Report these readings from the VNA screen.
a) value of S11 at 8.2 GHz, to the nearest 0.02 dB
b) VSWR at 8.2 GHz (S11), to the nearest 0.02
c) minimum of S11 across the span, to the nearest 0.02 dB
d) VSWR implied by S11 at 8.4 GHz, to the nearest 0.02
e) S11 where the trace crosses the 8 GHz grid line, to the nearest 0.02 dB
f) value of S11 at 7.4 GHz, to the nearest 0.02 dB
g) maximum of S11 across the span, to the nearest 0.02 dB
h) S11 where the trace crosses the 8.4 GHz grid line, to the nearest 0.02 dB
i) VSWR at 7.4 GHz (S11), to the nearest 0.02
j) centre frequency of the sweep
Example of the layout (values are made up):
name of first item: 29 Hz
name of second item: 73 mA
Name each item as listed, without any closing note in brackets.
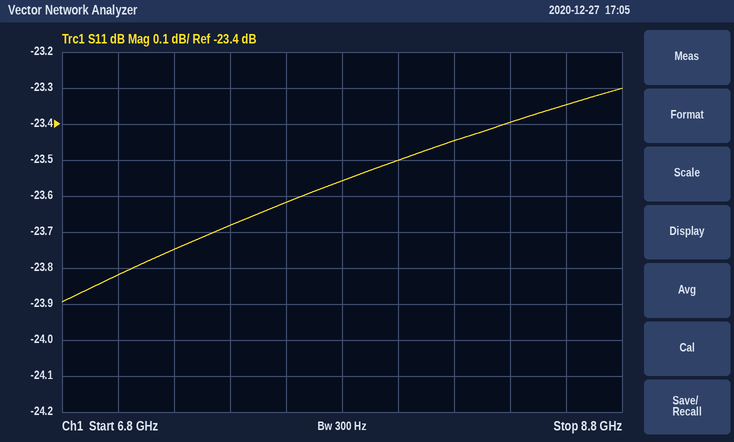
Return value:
value of S11 at 8.2 GHz, to the nearest 0.02 dB: -23.44 dB
VSWR at 8.2 GHz (S11), to the nearest 0.02: 1.14
minimum of S11 across the span, to the nearest 0.02 dB: -23.90 dB
VSWR implied by S11 at 8.4 GHz, to the nearest 0.02: 1.14
S11 where the trace crosses the 8 GHz grid line, to the nearest 0.02 dB: -23.50 dB
value of S11 at 7.4 GHz, to the nearest 0.02 dB: -23.68 dB
maximum of S11 across the span, to the nearest 0.02 dB: -23.30 dB
S11 where the trace crosses the 8.4 GHz grid line, to the nearest 0.02 dB: -23.40 dB
VSWR at 7.4 GHz (S11), to the nearest 0.02: 1.14
centre frequency of the sweep: 7.8 GHz
